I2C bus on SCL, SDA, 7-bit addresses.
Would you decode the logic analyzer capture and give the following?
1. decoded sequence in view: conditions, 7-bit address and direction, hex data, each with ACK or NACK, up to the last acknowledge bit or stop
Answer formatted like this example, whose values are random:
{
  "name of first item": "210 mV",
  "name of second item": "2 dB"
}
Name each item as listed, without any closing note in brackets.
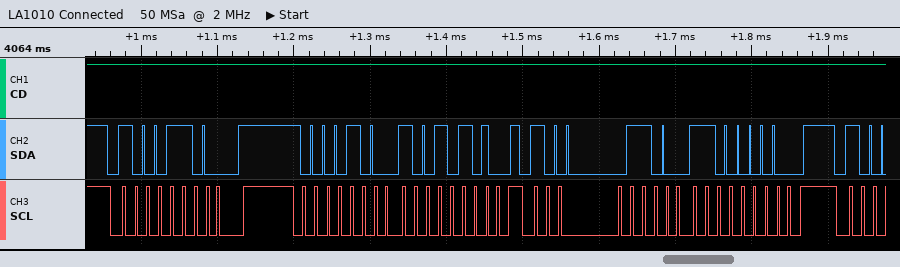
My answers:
{
  "decoded sequence in view: conditions, 7-bit address and direction, hex data, each with ACK or NACK, up to the last acknowledge bit or stop": "start, address 46 write ACK, 84 ACK, 95 ACK, stop, start, address 46 write ACK, C0 ACK, stop"
}
